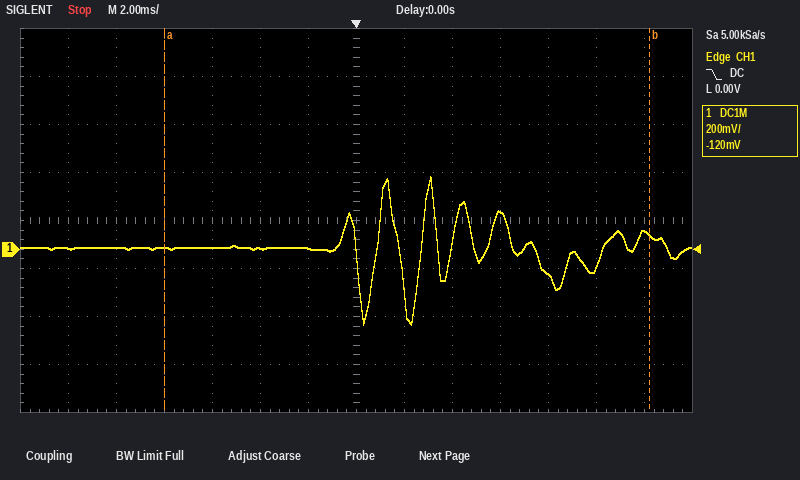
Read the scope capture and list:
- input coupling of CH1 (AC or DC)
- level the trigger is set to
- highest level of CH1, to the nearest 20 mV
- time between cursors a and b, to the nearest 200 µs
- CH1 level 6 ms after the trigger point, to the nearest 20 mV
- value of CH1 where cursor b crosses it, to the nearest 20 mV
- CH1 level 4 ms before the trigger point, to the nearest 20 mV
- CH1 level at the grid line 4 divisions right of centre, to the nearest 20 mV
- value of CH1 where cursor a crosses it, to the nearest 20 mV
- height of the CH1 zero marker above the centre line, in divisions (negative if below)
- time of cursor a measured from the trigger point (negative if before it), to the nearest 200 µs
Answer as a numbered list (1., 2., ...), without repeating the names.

1. DC
2. 0.00 V
3. 300 mV
4. 20.2 ms
5. 160 mV
6. 60 mV
7. 0 mV
8. -100 mV
9. 0 mV
10. -0.6 div
11. -8.0 ms
